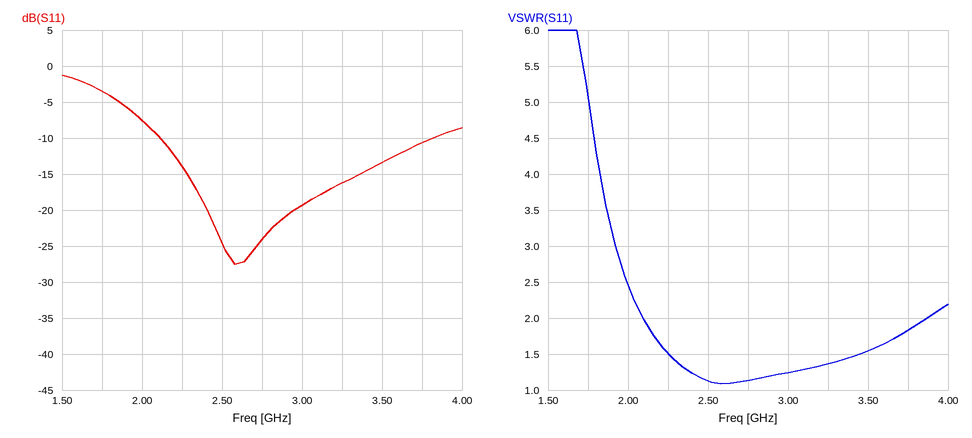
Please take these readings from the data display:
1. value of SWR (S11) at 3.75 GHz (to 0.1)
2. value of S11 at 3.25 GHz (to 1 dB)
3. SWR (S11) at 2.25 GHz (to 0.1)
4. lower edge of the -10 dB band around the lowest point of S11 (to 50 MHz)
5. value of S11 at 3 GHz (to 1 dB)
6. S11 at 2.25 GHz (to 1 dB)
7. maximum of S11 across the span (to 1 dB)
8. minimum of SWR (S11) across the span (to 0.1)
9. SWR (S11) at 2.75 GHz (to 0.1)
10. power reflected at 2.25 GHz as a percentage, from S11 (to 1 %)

1.8
-16 dB
1.5
2.10 GHz
-19 dB
-14 dB
-1 dB
1.1
1.1
4 %
